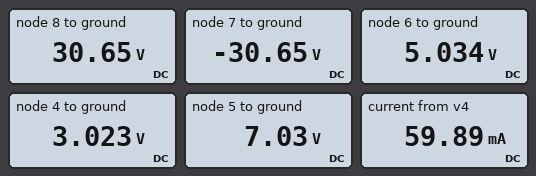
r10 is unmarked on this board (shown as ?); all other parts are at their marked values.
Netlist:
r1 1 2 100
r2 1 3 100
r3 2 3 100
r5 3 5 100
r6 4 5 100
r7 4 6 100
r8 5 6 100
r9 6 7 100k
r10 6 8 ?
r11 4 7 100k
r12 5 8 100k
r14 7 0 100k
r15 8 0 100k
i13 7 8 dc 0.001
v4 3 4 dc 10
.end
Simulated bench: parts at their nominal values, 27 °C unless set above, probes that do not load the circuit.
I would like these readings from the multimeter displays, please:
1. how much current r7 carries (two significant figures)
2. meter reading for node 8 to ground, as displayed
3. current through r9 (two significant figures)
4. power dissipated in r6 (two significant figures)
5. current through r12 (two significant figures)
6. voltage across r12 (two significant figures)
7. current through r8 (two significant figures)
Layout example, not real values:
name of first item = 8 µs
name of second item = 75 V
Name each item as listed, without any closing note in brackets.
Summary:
how much current r7 carries = 20 mA
meter reading for node 8 to ground, as displayed = 30.65 V
current through r9 = 360 µA
power dissipated in r6 = 160 mW
current through r12 = 240 µA
voltage across r12 = 24 V
current through r8 = 20 mA
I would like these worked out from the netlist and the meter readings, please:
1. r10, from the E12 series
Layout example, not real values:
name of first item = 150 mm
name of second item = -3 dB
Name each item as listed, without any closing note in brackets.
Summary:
r10, from the E12 series = 56 kΩ
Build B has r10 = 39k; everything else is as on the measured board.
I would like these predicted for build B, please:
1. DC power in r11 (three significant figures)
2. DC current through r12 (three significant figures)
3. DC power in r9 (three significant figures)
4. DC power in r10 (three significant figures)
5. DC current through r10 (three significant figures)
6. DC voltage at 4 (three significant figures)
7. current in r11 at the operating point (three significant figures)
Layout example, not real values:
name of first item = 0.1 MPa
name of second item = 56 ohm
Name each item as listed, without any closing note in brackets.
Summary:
DC power in r11 = 12.0 mW
DC current through r12 = 186 µA
DC power in r9 = 13.5 mW
DC power in r10 = 10.9 mW
DC current through r10 = 528 µA
DC voltage at 4 = 6.04 V
current in r11 at the operating point = 347 µA
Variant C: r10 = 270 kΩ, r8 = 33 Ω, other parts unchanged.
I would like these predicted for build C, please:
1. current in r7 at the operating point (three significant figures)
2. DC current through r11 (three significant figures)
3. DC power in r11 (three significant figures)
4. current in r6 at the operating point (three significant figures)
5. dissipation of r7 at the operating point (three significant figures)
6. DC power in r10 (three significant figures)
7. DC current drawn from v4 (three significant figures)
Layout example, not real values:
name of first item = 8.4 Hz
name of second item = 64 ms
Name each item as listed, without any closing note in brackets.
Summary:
current in r7 at the operating point = 27.4 mA
DC current through r11 = 293 µA
DC power in r11 = 8.57 mW
current in r6 at the operating point = 36.5 mA
dissipation of r7 at the operating point = 74.9 mW
DC power in r10 = 7.63 mW
DC current drawn from v4 = 63.5 mA
